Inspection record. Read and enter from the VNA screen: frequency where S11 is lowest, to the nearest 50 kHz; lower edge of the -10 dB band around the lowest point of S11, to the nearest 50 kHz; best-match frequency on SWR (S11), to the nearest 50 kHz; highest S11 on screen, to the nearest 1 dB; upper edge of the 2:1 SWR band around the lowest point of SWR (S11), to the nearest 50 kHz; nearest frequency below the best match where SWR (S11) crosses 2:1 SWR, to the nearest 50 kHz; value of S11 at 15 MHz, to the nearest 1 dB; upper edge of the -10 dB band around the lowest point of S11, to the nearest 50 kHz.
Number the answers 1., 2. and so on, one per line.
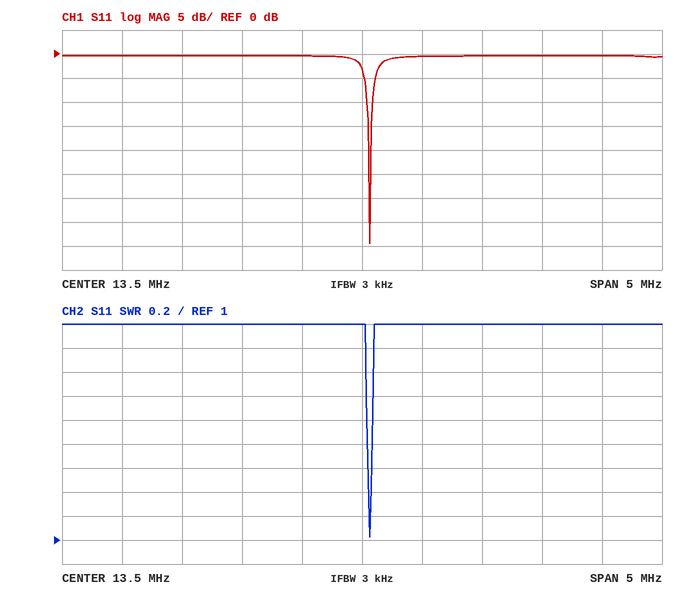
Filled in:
1. 13.55 MHz
2. 13.55 MHz
3. 13.55 MHz
4. 0 dB
5. 13.60 MHz
6. 13.55 MHz
7. 0 dB
8. 13.60 MHz
